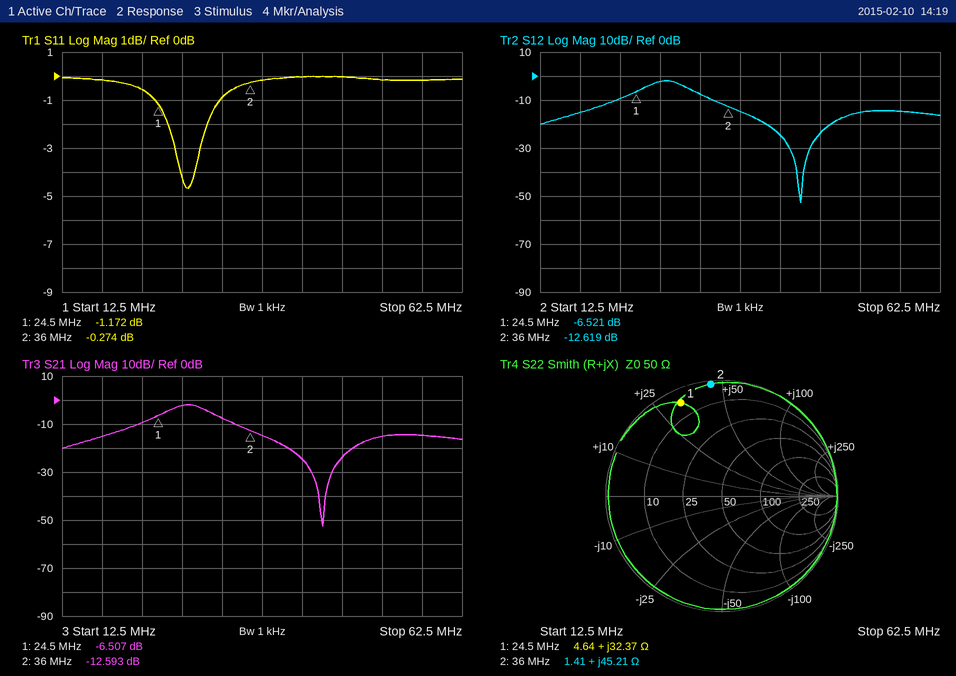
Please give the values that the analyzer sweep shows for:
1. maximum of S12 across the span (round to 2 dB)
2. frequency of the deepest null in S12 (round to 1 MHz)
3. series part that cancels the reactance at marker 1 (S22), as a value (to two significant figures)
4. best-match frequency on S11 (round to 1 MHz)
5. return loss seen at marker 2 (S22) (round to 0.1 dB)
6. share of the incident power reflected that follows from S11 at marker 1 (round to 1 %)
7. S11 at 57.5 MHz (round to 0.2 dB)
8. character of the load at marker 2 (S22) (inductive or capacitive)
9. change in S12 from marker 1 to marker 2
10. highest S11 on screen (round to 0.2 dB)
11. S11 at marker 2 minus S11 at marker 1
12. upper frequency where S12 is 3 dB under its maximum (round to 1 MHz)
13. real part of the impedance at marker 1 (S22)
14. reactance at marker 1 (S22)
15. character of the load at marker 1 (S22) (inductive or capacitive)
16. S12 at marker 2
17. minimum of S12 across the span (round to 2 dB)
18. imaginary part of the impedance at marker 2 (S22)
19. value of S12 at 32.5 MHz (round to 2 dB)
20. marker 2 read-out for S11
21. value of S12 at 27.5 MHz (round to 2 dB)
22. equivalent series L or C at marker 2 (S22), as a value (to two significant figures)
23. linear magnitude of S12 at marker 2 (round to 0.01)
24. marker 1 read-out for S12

-2 dB
45 MHz
200 pF
28 MHz
0.3 dB
76 %
-0.2 dB
inductive
-6.098 dB
0.0 dB
0.898 dB
31 MHz
4.64 Ω
+32.37 Ω
inductive
-12.619 dB
-52 dB
+45.21 Ω
-8 dB
-0.274 dB
-2 dB
200 nH
0.23
-6.521 dB
